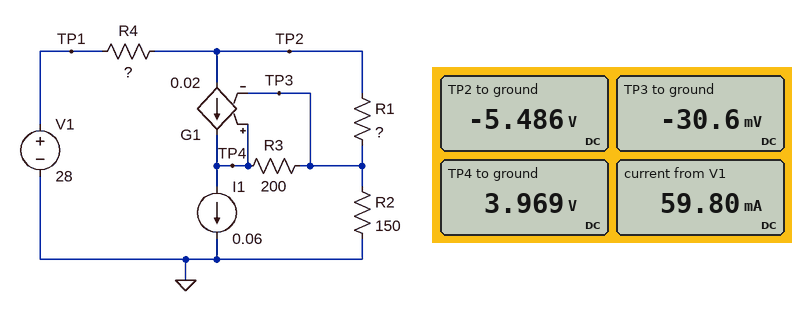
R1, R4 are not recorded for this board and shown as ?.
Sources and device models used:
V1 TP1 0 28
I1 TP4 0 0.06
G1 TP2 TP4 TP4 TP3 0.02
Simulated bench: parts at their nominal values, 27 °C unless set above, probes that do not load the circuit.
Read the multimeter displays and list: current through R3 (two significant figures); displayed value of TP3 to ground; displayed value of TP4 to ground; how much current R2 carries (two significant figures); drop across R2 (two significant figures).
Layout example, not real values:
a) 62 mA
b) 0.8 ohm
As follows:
a) 20 mA
b) -30.6 mV
c) 3.969 V
d) 200 µA
e) 31 mV
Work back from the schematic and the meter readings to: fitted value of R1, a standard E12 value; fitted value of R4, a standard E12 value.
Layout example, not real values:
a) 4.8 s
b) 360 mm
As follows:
a) 270 Ω
b) 560 Ω
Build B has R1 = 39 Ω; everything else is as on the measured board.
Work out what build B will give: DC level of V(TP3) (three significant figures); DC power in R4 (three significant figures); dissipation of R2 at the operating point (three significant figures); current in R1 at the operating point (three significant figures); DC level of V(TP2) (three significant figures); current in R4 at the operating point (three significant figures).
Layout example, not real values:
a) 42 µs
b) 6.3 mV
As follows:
a) -965 mV
b) 1.61 W
c) 6.21 mW
d) 26.4 mA
e) -2.00 V
f) 53.6 mA
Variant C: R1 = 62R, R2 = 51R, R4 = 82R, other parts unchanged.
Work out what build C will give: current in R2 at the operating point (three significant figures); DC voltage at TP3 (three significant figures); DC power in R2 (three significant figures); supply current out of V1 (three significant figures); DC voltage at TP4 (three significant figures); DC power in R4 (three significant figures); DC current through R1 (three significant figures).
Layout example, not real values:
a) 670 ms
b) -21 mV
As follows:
a) 125 mA
b) 6.36 V
c) 793 mW
d) 185 mA
e) 10.4 V
f) 2.80 W
g) 105 mA
